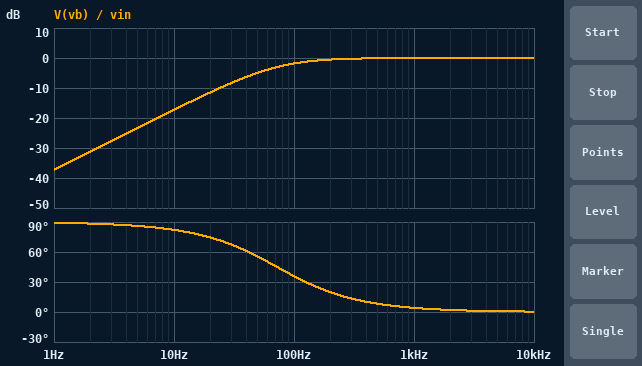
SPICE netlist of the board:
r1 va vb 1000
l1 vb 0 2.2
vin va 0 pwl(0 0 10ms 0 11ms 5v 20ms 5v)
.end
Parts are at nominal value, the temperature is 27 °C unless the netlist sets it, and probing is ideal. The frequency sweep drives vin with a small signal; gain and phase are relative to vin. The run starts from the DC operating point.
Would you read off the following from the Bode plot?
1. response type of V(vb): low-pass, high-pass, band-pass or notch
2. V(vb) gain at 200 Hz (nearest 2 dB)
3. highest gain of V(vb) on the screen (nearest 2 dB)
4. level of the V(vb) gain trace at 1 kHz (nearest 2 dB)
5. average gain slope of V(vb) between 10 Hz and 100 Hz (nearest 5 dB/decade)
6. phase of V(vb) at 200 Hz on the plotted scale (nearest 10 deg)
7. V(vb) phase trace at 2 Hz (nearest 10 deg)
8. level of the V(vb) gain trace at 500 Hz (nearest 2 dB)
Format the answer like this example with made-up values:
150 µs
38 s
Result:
high-pass
0 dB
0 dB
0 dB
15 dB/decade
20 deg
90 deg
0 dB
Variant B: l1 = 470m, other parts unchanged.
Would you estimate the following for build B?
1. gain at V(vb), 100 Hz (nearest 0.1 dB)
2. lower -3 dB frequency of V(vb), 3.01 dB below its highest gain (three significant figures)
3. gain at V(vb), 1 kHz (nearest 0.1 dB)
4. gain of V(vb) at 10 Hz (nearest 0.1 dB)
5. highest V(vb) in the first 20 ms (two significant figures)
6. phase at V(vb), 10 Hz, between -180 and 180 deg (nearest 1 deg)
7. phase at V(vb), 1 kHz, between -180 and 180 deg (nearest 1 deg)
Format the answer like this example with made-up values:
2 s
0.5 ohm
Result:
-11.0 dB
339 Hz
-0.5 dB
-30.6 dB
2.1 V
88 deg
19 deg
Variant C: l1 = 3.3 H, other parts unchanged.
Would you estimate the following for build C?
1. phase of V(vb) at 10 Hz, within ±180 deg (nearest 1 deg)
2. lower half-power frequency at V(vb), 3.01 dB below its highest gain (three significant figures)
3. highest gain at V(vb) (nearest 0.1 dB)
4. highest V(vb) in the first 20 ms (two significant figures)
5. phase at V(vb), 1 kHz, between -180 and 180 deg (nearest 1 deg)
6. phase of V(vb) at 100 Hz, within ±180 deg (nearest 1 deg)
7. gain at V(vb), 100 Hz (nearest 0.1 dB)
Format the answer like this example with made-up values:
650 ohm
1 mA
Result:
78 deg
48.2 Hz
0 dB
4.3 V
3 deg
26 deg
-0.9 dB
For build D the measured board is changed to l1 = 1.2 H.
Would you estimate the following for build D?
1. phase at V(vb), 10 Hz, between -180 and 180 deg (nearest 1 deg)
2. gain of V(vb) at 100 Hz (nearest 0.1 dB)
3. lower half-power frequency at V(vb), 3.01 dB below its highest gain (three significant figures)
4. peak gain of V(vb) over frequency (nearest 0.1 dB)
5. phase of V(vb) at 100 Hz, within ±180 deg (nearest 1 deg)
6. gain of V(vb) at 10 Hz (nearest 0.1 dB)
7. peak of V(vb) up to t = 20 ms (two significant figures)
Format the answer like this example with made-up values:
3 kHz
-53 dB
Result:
86 deg
-4.4 dB
133 Hz
0 dB
53 deg
-22.5 dB
3.4 V
